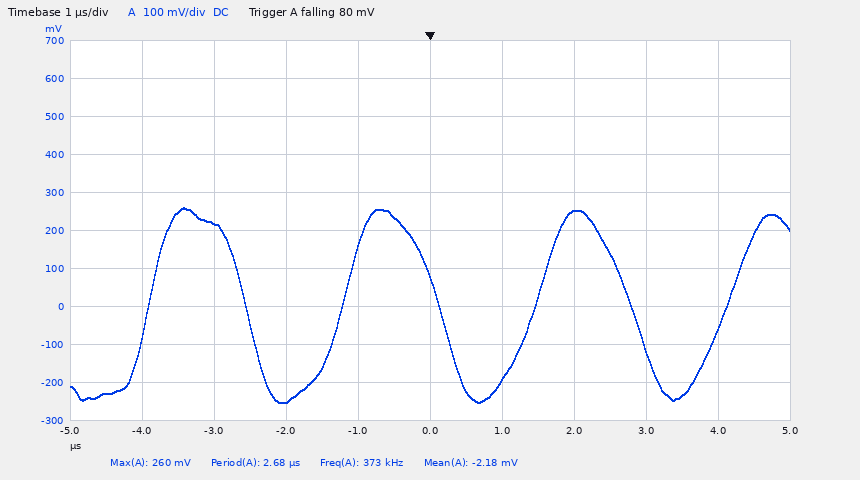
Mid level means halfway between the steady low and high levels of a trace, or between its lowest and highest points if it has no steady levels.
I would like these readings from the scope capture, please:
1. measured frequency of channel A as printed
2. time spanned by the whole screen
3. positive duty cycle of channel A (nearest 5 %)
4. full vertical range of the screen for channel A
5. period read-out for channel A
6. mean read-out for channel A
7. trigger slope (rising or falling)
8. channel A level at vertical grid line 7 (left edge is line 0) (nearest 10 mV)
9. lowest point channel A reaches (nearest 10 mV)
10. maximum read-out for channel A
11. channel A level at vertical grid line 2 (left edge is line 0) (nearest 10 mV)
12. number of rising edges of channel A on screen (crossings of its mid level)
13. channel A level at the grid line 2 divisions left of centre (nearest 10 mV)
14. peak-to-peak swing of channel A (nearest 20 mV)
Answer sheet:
373 kHz
10 µs
50 %
1 V
2.68 µs
-2.18 mV
falling
250 mV
-250 mV
260 mV
220 mV
4
-250 mV
520 mV
